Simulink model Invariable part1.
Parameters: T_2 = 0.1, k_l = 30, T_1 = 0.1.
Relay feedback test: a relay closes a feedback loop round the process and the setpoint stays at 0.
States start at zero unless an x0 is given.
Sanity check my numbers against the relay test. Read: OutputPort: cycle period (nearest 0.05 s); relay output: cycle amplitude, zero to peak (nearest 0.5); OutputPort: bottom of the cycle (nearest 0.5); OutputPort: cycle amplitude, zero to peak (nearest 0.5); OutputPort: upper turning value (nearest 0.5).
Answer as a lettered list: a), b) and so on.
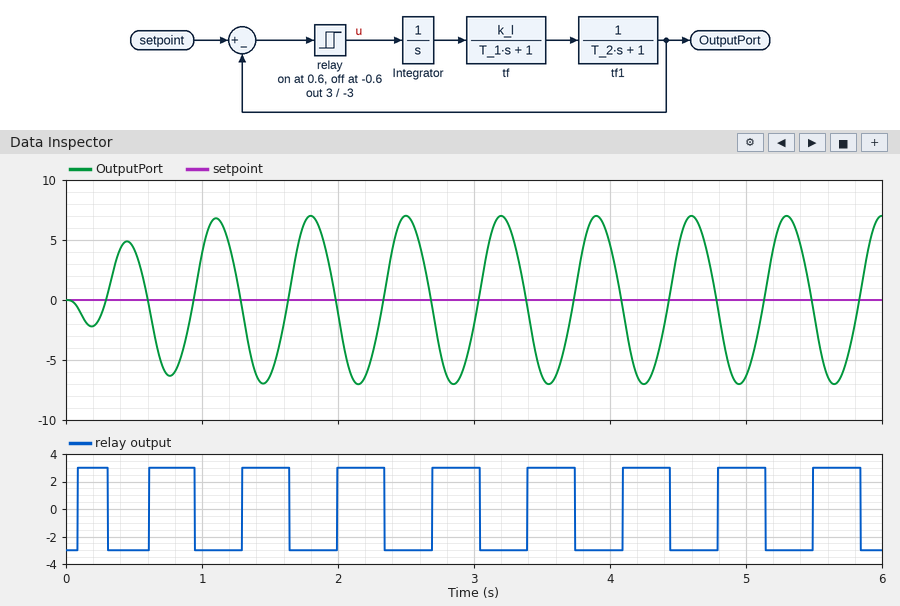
a) 0.70 s
b) 3.0
c) -7.0
d) 7.0
e) 7.0
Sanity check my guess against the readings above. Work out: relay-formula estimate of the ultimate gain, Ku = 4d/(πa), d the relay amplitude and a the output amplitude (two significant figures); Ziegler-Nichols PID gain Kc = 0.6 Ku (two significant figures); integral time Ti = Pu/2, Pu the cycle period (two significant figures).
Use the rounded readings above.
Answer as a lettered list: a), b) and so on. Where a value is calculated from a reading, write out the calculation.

a) 4 × 3 / (π × 7) = 0.55
b) 0.6 × 0.55 = 0.33
c) 0.7 / 2 = 0.35 s
